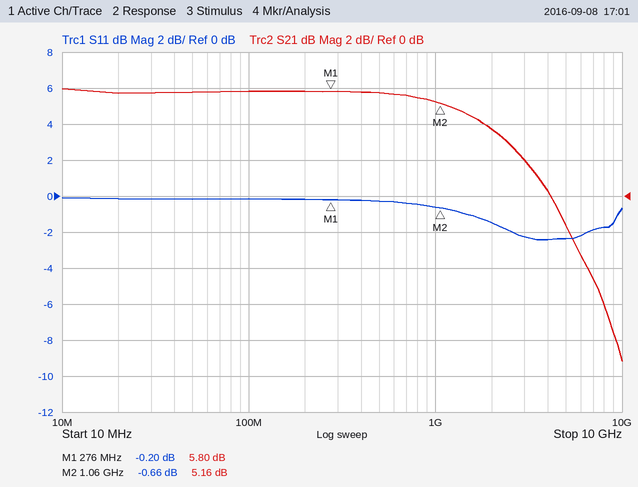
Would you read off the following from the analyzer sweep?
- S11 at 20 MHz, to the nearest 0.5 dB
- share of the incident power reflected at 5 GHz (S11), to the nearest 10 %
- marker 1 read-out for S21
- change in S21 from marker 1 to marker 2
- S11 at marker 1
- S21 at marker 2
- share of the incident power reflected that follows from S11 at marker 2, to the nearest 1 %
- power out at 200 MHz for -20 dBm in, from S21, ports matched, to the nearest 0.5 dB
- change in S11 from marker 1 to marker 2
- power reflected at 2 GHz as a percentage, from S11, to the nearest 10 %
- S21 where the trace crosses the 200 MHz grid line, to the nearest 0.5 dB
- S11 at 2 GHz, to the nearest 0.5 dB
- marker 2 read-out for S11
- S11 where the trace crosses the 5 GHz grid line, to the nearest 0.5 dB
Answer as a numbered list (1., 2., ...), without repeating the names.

1. 0.0 dB
2. 60 %
3. 5.80 dB
4. -0.64 dB
5. -0.20 dB
6. 5.16 dB
7. 86 %
8. -14.0 dBm
9. -0.46 dB
10. 70 %
11. 6.0 dB
12. -1.5 dB
13. -0.66 dB
14. -2.5 dB
